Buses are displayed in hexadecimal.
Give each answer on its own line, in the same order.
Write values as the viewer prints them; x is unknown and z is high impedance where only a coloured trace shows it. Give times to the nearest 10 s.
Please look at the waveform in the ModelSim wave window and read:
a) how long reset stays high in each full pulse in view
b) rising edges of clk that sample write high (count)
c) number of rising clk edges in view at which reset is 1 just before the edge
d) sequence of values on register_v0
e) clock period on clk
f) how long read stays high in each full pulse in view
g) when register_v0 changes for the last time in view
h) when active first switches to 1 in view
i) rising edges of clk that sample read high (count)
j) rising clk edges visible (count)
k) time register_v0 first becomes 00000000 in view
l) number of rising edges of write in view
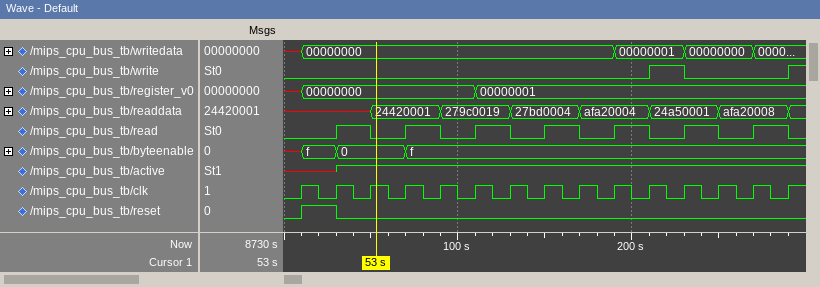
20 s
1
1
x, 00000000, 00000001
20 s
20 s, 20 s, 20 s, 20 s, 20 s, 20 s, 20 s
110 s
30 s
7
15
10 s
2
